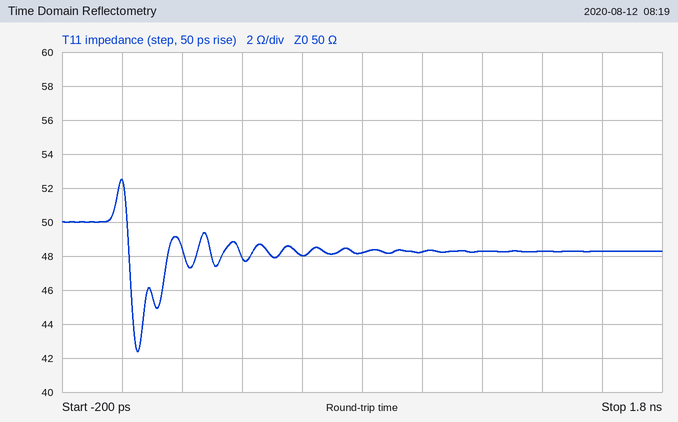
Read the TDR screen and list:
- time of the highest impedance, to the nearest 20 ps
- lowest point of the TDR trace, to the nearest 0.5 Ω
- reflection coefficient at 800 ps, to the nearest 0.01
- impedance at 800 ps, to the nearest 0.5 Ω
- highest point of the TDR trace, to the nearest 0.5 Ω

0 ps
42.5 Ω
-0.02
48.0 Ω
52.5 Ω
